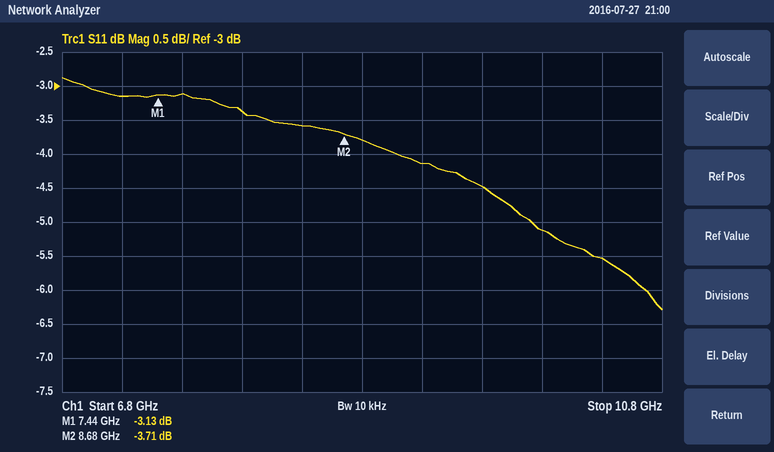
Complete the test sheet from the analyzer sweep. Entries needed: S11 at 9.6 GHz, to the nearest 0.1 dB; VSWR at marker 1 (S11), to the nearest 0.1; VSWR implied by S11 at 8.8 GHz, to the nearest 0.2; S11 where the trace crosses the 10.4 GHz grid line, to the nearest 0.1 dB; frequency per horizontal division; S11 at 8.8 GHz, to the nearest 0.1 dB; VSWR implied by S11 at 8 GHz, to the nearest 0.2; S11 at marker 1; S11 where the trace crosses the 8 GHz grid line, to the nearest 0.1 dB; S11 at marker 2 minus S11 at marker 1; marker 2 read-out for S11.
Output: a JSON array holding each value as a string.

["-4.5 dB", "5.6", "4.6", "-5.5 dB", "400 MHz", "-3.8 dB", "5.2", "-3.13 dB", "-3.4 dB", "-0.58 dB", "-3.71 dB"]
